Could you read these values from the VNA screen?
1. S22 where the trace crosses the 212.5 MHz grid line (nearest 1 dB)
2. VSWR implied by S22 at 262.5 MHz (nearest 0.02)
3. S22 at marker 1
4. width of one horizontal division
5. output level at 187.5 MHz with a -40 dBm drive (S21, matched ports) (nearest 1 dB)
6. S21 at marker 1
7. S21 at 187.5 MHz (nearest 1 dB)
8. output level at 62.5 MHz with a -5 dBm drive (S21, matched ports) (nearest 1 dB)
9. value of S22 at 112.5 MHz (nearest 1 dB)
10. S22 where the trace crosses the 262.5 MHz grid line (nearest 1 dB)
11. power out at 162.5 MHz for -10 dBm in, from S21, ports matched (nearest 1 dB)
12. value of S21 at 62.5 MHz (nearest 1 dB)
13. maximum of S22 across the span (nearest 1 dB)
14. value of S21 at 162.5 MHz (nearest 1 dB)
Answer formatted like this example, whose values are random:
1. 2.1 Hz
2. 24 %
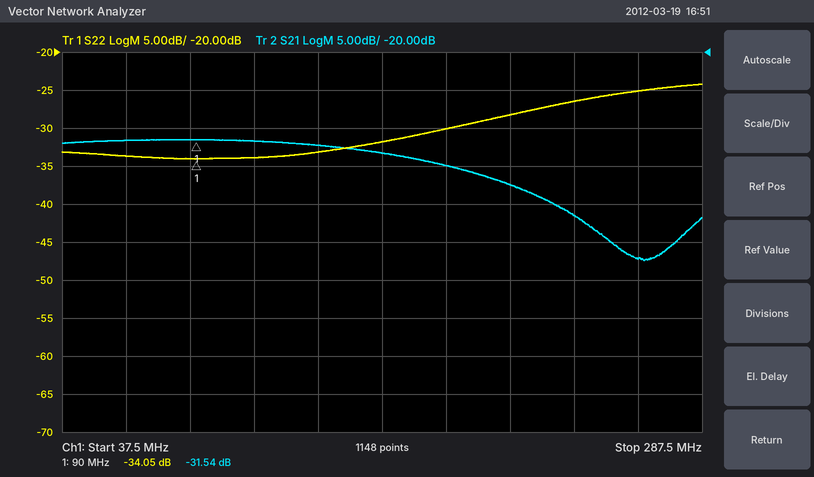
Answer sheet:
1. -28 dB
2. 1.12
3. -34.05 dB
4. 25 MHz
5. -75 dBm
6. -31.54 dB
7. -35 dB
8. -37 dBm
9. -34 dB
10. -25 dB
11. -43 dBm
12. -32 dB
13. -24 dB
14. -33 dB
